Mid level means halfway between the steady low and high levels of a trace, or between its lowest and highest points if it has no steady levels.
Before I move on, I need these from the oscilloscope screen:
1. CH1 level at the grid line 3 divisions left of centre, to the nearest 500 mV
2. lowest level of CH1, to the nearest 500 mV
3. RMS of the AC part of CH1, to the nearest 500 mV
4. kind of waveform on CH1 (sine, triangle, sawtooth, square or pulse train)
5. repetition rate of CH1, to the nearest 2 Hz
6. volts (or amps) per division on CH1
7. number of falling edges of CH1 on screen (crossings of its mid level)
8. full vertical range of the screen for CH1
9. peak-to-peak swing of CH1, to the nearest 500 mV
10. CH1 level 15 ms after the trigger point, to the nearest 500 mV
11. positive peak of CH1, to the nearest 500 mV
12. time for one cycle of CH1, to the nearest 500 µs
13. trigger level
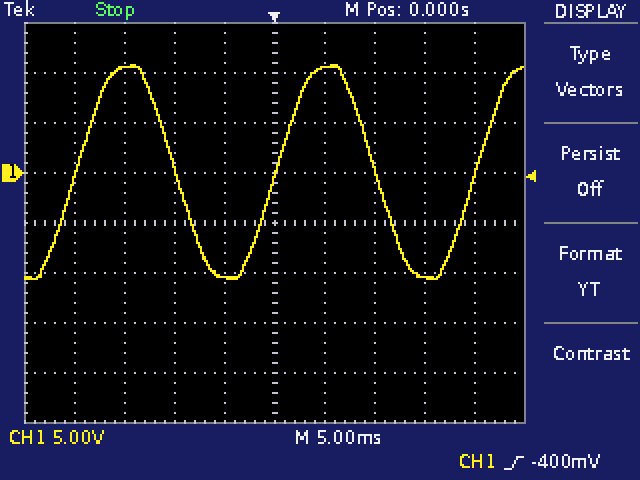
10.5 V
-10.5 V
7.5 V
sine
50 Hz
5 V
2
40 V
21.5 V
-10.5 V
11.0 V
20.0 ms
-400 mV
